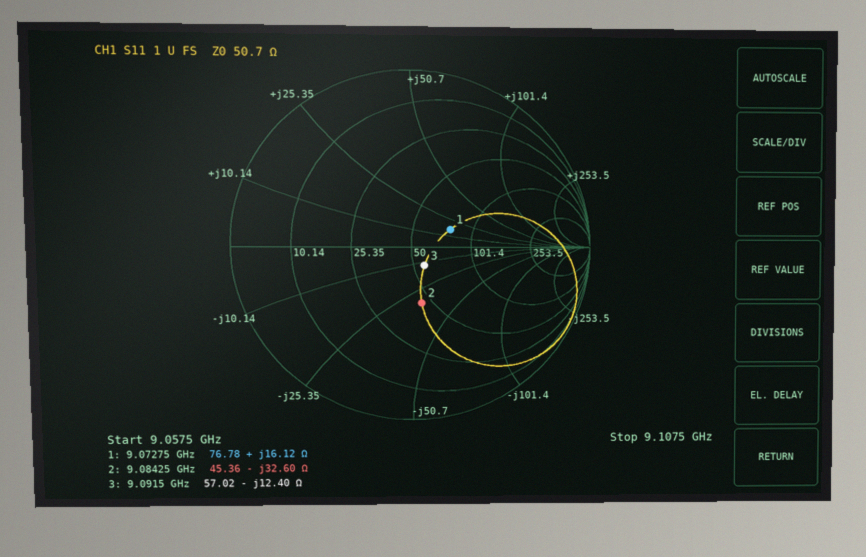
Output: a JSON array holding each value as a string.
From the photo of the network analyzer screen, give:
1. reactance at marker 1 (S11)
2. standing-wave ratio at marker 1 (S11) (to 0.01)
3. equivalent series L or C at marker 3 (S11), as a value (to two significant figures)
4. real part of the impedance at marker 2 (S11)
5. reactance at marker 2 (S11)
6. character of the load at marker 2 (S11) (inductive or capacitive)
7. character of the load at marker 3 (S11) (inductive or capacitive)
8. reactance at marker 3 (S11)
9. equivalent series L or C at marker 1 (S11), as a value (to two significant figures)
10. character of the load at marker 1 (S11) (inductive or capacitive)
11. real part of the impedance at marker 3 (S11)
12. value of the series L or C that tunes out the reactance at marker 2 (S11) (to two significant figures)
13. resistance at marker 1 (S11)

["+16.12 Ω", "1.63", "1.4 pF", "45.36 Ω", "-32.60 Ω", "capacitive", "capacitive", "-12.40 Ω", "280 pH", "inductive", "57.02 Ω", "570 pH", "76.78 Ω"]
